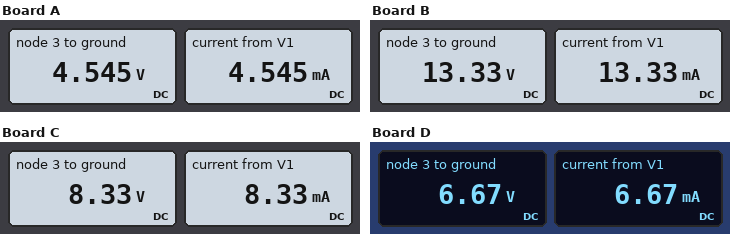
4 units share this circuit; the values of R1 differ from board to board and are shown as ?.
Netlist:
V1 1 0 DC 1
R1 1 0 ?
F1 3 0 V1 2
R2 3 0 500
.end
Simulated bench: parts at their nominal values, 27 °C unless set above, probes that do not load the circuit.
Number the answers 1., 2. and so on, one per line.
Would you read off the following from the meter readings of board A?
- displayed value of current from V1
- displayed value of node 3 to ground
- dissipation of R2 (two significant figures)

1. 4.545 mA
2. 4.545 V
3. 41 mW
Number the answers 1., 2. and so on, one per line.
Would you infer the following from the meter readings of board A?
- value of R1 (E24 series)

1. 220 Ω
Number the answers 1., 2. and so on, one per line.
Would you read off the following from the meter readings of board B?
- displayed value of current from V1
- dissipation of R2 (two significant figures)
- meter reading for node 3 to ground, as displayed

1. 13.33 mA
2. 360 mW
3. 13.33 V
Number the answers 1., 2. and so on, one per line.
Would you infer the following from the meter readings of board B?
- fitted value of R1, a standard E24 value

1. 75 Ω
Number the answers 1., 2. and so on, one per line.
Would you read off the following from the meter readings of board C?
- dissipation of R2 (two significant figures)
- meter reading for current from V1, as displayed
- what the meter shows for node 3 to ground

1. 140 mW
2. 8.33 mA
3. 8.33 V
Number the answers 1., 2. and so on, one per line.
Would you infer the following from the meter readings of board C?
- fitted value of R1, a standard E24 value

1. 120 Ω
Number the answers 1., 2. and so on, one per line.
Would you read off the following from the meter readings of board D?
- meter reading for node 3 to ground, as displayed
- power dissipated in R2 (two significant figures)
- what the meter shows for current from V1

1. 6.67 V
2. 89 mW
3. 6.67 mA
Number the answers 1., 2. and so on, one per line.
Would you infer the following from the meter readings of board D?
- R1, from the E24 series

1. 150 Ω
